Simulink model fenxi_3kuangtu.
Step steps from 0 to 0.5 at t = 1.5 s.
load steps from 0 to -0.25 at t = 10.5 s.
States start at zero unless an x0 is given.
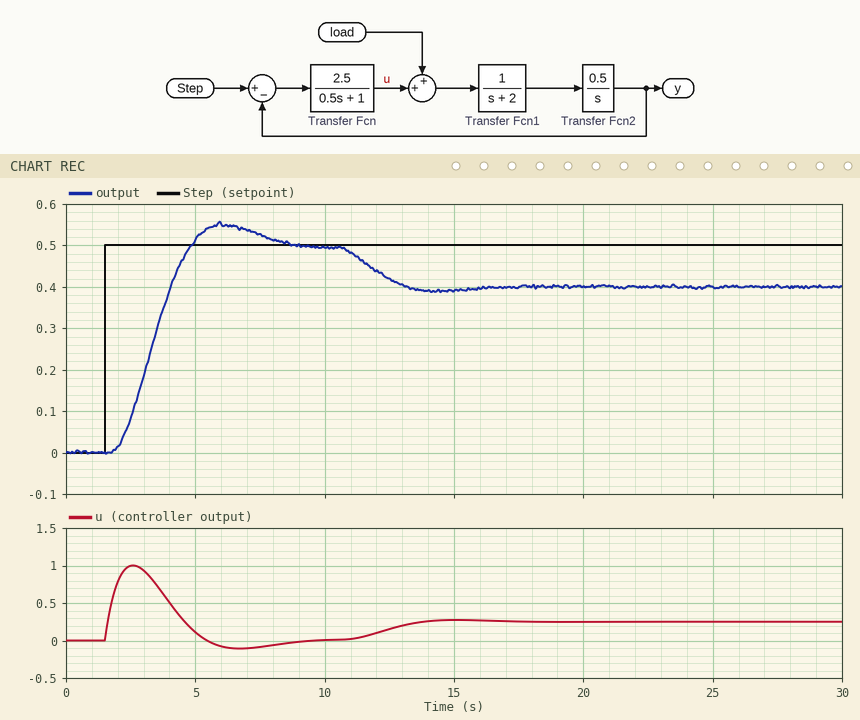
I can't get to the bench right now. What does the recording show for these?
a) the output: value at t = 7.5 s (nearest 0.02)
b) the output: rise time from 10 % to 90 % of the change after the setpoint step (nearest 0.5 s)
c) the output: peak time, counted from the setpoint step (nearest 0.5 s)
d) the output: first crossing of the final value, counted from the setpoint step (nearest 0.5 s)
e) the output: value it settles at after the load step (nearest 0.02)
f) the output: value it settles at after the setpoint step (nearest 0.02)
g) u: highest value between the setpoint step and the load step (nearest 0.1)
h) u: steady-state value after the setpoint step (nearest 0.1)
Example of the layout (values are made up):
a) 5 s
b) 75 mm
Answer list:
a) 0.52
b) 2.0 s
c) 4.5 s
d) 3.5 s
e) 0.40
f) 0.50
g) 1.0
h) 0.0
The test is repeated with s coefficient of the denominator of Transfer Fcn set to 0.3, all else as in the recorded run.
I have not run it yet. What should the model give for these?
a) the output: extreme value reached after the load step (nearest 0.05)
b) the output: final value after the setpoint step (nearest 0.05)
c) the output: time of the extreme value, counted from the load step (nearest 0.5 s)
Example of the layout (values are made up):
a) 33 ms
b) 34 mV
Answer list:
a) 0.40
b) 0.50
c) 4.0 s
